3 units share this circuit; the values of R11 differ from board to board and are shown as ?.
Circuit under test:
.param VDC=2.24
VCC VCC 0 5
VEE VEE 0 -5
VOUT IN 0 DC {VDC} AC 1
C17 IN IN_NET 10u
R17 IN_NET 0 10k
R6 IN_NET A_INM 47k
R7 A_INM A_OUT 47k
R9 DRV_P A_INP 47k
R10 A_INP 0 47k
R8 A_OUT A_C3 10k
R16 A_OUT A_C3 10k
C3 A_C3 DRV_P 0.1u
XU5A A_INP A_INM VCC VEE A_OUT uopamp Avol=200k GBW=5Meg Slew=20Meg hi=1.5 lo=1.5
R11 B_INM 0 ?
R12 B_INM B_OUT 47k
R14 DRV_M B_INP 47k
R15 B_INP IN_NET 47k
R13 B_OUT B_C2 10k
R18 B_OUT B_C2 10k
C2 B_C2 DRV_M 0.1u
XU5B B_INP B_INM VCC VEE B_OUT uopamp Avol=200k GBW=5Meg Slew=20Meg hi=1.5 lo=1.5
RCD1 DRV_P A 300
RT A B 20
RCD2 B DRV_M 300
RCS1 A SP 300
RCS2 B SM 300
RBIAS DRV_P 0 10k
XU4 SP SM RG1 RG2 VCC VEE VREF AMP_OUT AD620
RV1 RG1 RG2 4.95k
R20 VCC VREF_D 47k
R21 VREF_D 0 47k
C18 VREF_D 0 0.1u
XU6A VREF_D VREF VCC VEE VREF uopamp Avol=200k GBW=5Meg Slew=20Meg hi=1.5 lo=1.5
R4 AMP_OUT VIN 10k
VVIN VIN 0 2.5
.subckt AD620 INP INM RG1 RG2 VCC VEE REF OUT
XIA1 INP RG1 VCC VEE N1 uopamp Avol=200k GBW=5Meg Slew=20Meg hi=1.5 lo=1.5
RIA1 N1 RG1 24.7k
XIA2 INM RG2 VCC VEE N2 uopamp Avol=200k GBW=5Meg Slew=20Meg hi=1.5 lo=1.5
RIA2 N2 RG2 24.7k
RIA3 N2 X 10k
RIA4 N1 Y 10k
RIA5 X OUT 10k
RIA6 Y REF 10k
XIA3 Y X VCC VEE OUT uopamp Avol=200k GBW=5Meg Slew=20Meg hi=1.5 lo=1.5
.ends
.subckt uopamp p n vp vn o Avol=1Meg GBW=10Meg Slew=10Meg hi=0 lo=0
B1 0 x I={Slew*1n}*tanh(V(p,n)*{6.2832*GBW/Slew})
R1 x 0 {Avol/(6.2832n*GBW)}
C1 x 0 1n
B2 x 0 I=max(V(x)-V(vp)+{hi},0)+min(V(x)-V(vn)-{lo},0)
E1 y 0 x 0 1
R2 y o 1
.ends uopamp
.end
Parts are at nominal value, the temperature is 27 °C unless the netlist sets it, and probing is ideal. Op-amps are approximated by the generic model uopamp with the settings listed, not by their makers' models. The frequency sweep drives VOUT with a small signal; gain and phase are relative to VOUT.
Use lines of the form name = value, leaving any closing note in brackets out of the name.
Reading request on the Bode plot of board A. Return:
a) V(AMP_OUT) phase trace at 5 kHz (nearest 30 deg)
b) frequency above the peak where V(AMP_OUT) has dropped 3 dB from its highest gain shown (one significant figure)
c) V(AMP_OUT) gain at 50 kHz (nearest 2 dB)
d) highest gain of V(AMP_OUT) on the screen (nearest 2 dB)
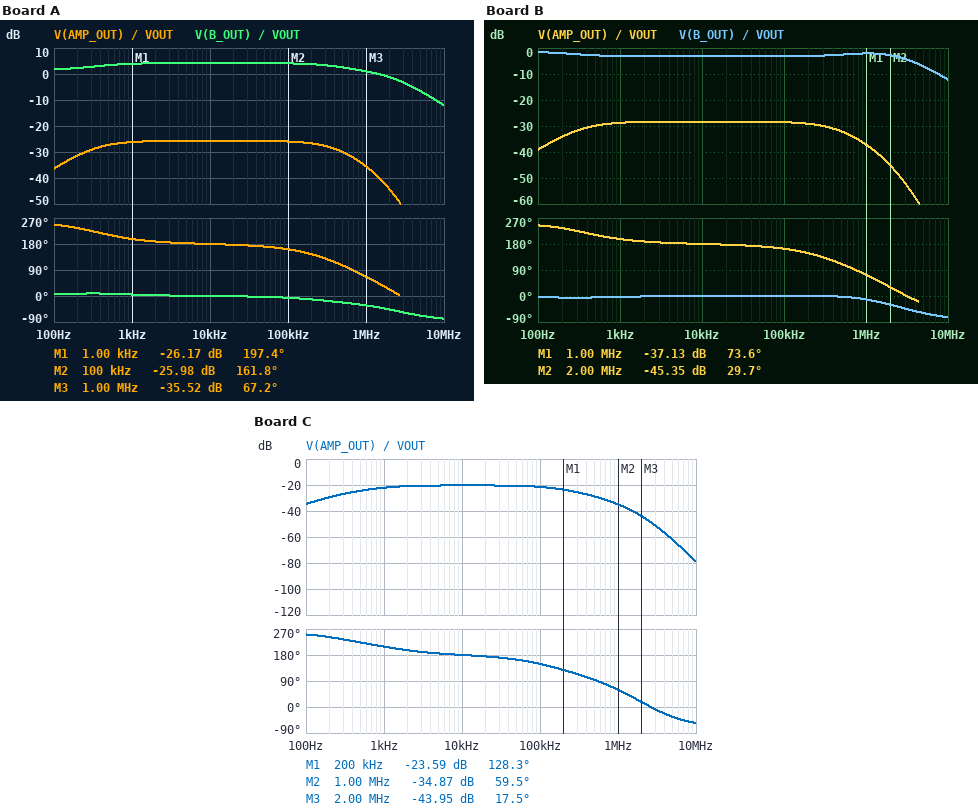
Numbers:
V(AMP_OUT) phase trace at 5 kHz = 180 deg
frequency above the peak where V(AMP_OUT) has dropped 3 dB from its highest gain shown = 400 kHz
V(AMP_OUT) gain at 50 kHz = -26 dB
highest gain of V(AMP_OUT) on the screen = -26 dB
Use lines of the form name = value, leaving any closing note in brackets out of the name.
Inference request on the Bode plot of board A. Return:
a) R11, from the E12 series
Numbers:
R11, from the E12 series = 39 kΩ
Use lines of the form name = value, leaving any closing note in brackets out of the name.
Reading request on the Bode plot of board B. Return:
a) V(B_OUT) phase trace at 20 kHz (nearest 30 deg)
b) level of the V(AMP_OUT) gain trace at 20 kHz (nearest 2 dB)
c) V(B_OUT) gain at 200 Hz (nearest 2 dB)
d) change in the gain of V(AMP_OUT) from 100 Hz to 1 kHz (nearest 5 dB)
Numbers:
V(B_OUT) phase trace at 20 kHz = 0 deg
level of the V(AMP_OUT) gain trace at 20 kHz = -28 dB
V(B_OUT) gain at 200 Hz = -2 dB
change in the gain of V(AMP_OUT) from 100 Hz to 1 kHz = 10 dB
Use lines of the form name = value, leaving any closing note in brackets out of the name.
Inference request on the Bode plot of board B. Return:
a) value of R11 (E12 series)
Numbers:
value of R11 = 82 kΩ
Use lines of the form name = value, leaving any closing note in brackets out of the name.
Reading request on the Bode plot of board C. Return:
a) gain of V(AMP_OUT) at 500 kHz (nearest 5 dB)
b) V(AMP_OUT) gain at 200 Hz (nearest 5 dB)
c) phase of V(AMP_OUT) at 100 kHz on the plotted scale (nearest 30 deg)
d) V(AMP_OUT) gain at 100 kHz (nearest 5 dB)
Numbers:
gain of V(AMP_OUT) at 500 kHz = -30 dB
V(AMP_OUT) gain at 200 Hz = -30 dB
phase of V(AMP_OUT) at 100 kHz on the plotted scale = 150 deg
V(AMP_OUT) gain at 100 kHz = -20 dB
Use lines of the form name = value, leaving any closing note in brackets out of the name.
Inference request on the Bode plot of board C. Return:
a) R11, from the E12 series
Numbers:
R11, from the E12 series = 27 kΩ
